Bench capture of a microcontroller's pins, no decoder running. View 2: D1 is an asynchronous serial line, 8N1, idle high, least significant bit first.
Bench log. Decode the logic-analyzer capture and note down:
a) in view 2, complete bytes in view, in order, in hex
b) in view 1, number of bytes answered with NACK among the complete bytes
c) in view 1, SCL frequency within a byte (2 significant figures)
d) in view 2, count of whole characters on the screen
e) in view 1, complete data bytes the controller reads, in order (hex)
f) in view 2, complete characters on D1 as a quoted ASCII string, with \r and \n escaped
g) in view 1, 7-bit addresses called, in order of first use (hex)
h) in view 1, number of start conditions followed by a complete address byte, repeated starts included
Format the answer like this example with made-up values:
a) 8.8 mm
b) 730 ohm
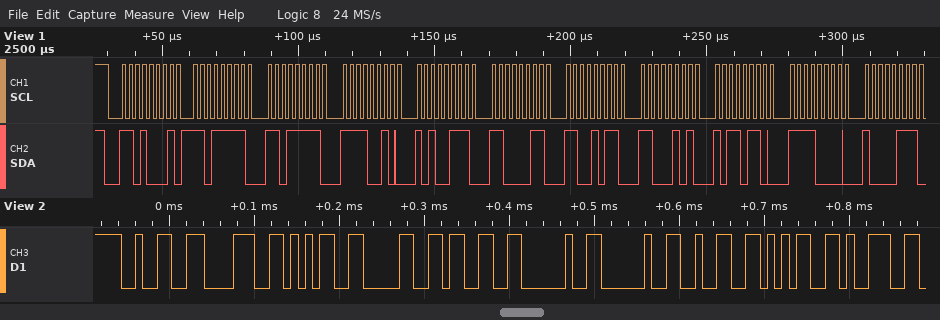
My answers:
a) 32 38 35 30 33 20 20 32 35 39
b) 0
c) 400 kHz
d) 10
e) DF DF F2 A7 C3 CB C5 B6 F0 87
f) "28503  259"
g) 0x68
h) 1
